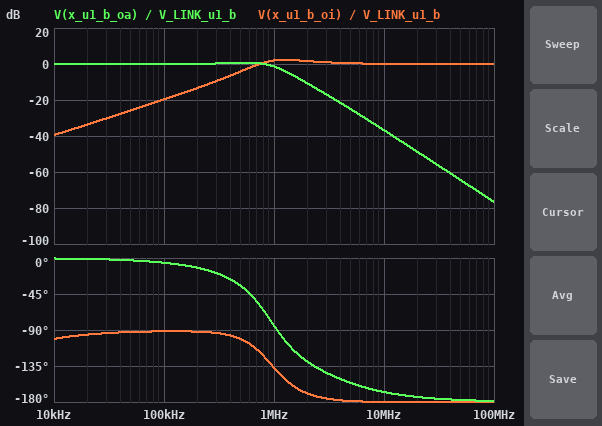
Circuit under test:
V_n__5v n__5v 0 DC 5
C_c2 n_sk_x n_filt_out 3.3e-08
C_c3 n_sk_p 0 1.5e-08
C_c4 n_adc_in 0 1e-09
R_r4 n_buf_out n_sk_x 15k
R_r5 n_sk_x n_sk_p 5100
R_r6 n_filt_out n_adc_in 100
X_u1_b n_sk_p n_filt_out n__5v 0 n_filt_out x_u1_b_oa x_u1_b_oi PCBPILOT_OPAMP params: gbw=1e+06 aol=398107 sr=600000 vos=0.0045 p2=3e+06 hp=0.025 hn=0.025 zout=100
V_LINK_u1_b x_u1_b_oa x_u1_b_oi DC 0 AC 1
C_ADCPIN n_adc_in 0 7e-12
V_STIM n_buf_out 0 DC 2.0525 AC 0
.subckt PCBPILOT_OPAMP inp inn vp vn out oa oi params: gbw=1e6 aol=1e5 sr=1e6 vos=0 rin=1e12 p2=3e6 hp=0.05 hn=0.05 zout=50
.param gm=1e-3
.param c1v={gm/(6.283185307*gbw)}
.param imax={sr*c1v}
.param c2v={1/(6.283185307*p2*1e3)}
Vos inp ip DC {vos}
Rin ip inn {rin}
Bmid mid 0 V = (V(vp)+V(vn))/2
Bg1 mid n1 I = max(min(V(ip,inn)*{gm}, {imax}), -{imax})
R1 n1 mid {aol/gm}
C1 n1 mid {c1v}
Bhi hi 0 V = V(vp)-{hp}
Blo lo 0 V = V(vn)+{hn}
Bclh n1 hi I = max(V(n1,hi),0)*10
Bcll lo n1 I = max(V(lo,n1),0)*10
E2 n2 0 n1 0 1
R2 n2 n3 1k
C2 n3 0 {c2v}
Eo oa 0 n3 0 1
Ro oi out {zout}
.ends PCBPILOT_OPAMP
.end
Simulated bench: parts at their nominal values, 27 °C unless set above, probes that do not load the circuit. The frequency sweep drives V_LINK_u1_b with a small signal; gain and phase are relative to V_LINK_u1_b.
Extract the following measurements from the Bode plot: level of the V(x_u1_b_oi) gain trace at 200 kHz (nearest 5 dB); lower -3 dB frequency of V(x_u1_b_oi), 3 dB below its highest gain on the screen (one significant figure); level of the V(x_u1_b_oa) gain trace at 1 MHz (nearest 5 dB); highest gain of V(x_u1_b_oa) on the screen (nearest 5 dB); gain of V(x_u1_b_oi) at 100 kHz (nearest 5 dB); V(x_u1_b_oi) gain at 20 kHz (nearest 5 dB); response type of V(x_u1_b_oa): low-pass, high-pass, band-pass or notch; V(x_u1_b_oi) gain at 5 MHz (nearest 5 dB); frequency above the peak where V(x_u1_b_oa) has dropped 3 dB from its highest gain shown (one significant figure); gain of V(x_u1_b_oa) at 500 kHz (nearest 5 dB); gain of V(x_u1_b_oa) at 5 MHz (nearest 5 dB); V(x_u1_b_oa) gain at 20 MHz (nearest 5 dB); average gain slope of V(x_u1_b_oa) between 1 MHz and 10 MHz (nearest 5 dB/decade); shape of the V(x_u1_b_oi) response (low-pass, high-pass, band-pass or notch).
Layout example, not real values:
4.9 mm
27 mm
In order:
-15 dB
700 kHz
0 dB
0 dB
-20 dB
-35 dB
low-pass
0 dB
1 MHz
0 dB
-25 dB
-50 dB
-35 dB/decade
high-pass
